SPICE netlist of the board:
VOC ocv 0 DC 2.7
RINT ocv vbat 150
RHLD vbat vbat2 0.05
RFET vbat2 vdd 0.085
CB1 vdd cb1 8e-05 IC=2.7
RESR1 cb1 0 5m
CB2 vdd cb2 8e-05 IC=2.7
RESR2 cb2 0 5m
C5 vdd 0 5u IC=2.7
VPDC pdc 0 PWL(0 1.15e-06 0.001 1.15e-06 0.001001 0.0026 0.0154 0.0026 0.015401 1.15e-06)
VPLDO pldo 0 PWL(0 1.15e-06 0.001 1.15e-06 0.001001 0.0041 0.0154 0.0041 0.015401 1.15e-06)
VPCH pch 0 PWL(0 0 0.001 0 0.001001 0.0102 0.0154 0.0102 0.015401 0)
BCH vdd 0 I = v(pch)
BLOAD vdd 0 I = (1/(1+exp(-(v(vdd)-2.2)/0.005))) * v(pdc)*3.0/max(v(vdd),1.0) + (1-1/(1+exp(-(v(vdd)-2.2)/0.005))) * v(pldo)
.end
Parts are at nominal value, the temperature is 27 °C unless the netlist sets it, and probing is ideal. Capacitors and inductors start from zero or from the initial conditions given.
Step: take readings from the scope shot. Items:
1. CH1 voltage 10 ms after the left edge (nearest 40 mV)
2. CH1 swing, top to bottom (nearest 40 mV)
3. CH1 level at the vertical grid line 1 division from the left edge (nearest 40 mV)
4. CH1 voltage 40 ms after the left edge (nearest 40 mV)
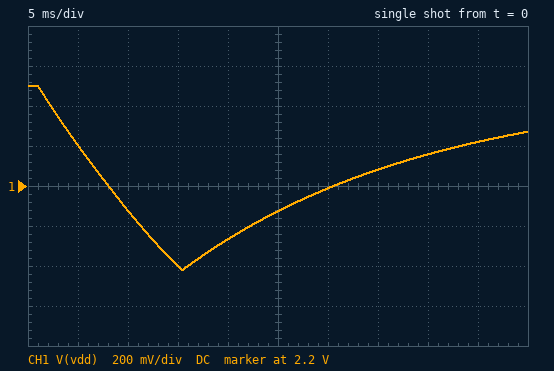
2.08 V
920 mV
2.40 V
2.36 V
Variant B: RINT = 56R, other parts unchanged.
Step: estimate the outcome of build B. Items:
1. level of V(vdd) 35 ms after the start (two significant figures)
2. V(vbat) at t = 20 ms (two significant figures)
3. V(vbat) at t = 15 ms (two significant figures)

2.6 V
2.3 V
2.1 V
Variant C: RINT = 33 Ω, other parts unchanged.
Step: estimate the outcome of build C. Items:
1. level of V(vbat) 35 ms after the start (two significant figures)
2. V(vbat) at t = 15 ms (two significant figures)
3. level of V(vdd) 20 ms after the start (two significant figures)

2.7 V
2.3 V
2.5 V
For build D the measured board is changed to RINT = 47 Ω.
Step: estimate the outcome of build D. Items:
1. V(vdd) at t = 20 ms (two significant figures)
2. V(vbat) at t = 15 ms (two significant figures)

2.4 V
2.2 V
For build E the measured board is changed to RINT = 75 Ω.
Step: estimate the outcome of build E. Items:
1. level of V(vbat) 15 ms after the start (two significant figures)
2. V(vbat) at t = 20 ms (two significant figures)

2.0 V
2.2 V
